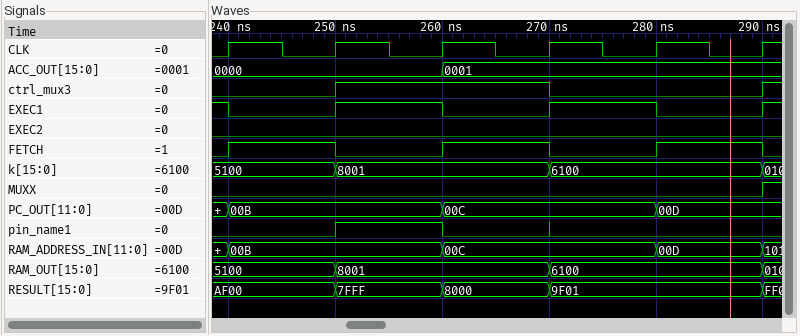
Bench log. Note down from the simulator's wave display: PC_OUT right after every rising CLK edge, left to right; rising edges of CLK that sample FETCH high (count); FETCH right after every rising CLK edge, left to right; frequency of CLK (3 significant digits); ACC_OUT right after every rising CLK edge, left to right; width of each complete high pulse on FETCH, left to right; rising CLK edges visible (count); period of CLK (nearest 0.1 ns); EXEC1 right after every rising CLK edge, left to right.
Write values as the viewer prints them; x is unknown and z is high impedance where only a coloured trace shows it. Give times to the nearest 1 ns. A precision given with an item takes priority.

00B, 00B, 00C, 00C, 00D, 00D
3
1 0 1 0 1 0
100 MHz
0000, 0000, 0001, 0001, 0001, 0001
10 ns, 10 ns, 10 ns
6
10 ns
0 1 0 1 0 1
